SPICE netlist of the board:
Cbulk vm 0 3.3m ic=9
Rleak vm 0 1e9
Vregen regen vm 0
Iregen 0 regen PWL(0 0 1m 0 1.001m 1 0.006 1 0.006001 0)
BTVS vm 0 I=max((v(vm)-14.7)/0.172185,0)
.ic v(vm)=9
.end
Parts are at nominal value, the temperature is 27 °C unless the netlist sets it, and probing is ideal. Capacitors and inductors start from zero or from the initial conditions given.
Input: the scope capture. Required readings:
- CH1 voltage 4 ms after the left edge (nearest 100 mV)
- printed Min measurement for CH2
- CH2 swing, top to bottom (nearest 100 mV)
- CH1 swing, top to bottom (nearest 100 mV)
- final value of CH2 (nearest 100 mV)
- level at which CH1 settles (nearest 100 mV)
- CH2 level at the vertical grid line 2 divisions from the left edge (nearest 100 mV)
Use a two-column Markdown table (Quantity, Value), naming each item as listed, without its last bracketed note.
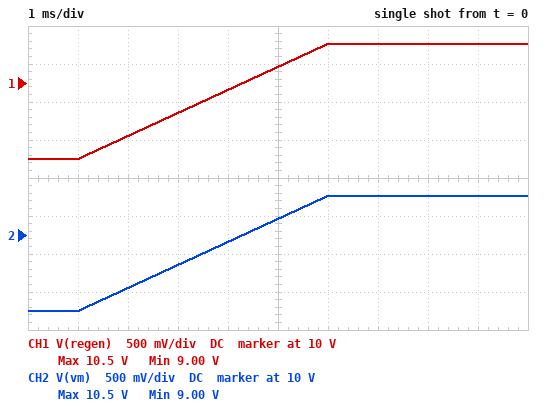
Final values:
| Quantity | Value |
|---|---|
| CH1 voltage 4 ms after the left edge | 9.9 V |
| printed Min measurement for CH2 | 9.00 V |
| CH2 swing, top to bottom | 1.5 V |
| CH1 swing, top to bottom | 1.5 V |
| final value of CH2 | 10.5 V |
| level at which CH1 settles | 10.5 V |
| CH2 level at the vertical grid line 2 divisions from the left edge | 9.3 V |
